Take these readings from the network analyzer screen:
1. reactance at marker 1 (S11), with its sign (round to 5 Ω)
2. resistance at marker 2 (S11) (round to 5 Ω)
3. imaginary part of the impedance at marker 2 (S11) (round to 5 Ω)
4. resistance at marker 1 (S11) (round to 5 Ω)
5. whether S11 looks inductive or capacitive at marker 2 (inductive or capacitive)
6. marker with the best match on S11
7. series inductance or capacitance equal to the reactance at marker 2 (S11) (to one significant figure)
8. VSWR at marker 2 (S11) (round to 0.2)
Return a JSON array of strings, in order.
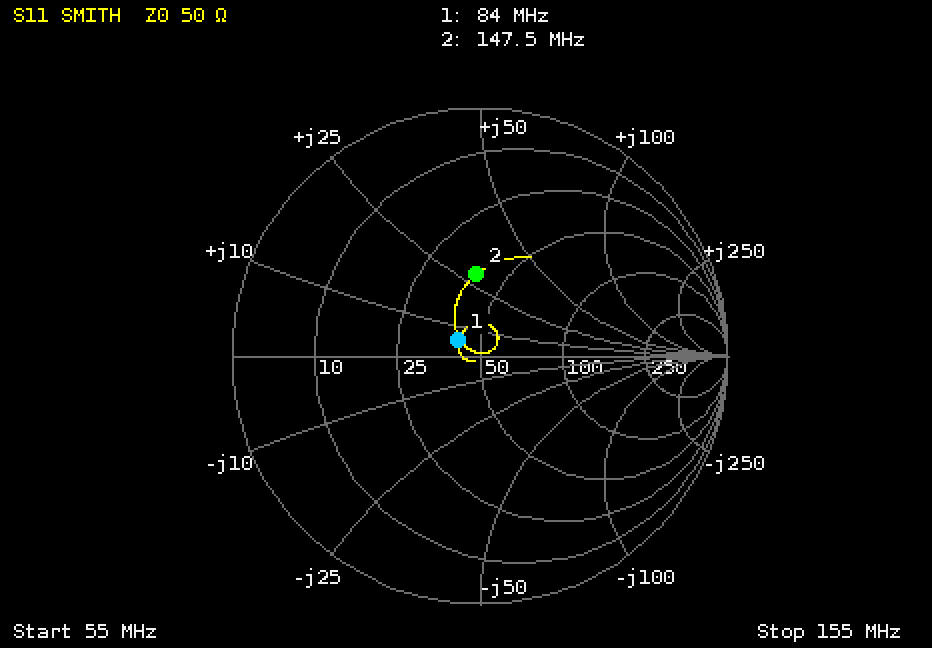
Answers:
["+5 Ω", "40 Ω", "+30 Ω", "40 Ω", "inductive", "marker 1", "30 nH", "2.0"]
